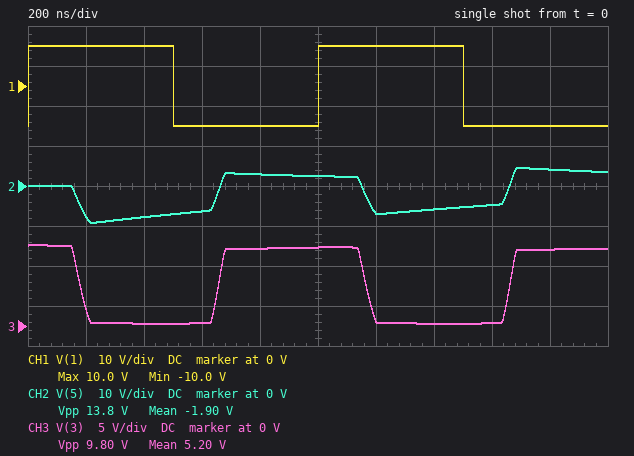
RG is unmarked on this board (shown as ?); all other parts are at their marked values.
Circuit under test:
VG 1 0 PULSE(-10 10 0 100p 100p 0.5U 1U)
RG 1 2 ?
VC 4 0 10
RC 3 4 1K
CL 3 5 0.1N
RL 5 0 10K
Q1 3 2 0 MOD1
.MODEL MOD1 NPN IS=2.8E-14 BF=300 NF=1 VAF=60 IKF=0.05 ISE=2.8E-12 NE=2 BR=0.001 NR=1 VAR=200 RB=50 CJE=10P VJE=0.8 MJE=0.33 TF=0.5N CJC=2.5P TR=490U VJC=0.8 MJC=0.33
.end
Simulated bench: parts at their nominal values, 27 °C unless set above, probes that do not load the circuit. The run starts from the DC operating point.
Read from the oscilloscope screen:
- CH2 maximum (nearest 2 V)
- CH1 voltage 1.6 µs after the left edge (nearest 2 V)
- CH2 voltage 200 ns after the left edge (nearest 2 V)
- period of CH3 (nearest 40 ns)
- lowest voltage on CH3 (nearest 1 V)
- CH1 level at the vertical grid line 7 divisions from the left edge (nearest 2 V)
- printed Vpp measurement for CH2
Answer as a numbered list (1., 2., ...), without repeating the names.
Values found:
1. 4 V
2. -10 V
3. -8 V
4. 1.00 µs
5. 0 V
6. 10 V
7. 13.8 V
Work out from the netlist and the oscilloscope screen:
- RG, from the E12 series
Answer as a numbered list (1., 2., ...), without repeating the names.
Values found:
1. 27 kΩ
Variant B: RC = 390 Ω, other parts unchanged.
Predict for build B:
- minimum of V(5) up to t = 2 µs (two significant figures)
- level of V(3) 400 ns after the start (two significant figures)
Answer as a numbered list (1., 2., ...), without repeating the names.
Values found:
1. -9.0 V
2. 350 mV
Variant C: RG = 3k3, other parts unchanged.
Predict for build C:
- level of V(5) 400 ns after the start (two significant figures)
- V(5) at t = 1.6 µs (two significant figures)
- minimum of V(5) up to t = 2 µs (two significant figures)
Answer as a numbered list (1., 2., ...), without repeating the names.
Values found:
1. -6.7 V
2. -3.4 V
3. -9.6 V
